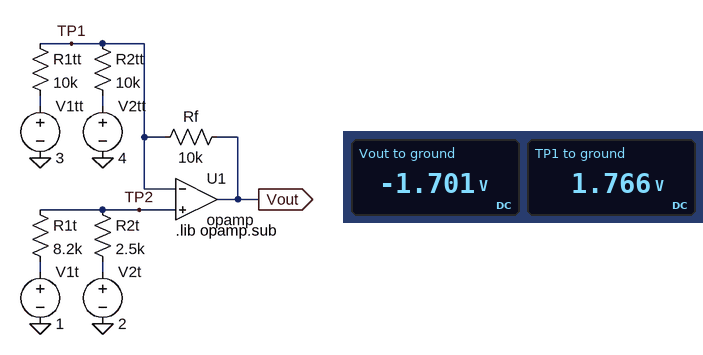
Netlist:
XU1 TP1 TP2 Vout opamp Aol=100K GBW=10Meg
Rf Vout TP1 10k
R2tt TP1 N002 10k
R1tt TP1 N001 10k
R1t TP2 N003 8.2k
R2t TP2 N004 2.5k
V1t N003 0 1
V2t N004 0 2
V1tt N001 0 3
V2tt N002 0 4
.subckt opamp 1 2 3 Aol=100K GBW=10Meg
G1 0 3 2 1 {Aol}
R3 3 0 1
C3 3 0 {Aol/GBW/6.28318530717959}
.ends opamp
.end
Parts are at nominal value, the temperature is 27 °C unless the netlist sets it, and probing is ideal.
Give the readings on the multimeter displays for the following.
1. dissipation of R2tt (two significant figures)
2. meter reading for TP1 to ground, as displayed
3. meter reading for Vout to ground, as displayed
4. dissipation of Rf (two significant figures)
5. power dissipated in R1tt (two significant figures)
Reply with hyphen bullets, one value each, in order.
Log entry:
- 500 µW
- 1.766 V
- -1.701 V
- 1.2 mW
- 150 µW
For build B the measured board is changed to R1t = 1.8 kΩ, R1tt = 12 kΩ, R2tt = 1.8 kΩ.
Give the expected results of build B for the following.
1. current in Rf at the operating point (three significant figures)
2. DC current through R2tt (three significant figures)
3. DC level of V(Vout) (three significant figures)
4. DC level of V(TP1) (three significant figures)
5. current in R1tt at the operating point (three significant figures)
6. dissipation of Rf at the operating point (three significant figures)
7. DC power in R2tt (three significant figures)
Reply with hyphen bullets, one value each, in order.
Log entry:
- 1.57 mA
- 1.43 mA
- -14.2 V
- 1.42 V
- 132 µA
- 24.5 mW
- 3.70 mW
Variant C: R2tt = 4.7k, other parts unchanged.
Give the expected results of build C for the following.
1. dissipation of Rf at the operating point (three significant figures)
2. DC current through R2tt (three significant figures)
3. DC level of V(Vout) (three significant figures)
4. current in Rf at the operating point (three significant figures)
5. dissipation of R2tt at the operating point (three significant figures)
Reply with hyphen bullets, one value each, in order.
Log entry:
- 3.58 mW
- 475 µA
- -4.22 V
- 599 µA
- 1.06 mW
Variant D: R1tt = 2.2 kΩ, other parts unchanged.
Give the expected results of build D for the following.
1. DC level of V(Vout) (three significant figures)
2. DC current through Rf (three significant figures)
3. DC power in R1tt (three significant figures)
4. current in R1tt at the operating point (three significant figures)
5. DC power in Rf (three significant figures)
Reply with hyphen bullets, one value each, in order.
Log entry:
- -6.07 V
- 784 µA
- 692 µW
- 561 µA
- 6.15 mW
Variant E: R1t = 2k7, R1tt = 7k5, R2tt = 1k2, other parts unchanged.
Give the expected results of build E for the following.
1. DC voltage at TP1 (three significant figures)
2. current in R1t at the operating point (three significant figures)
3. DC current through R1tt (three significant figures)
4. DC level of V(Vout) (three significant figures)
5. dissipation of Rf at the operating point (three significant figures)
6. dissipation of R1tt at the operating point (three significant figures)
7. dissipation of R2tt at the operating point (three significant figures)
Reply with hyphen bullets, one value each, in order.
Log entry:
- 1.52 V
- 192 µA
- 197 µA
- -21.1 V
- 51.3 mW
- 292 µW
- 5.13 mW
